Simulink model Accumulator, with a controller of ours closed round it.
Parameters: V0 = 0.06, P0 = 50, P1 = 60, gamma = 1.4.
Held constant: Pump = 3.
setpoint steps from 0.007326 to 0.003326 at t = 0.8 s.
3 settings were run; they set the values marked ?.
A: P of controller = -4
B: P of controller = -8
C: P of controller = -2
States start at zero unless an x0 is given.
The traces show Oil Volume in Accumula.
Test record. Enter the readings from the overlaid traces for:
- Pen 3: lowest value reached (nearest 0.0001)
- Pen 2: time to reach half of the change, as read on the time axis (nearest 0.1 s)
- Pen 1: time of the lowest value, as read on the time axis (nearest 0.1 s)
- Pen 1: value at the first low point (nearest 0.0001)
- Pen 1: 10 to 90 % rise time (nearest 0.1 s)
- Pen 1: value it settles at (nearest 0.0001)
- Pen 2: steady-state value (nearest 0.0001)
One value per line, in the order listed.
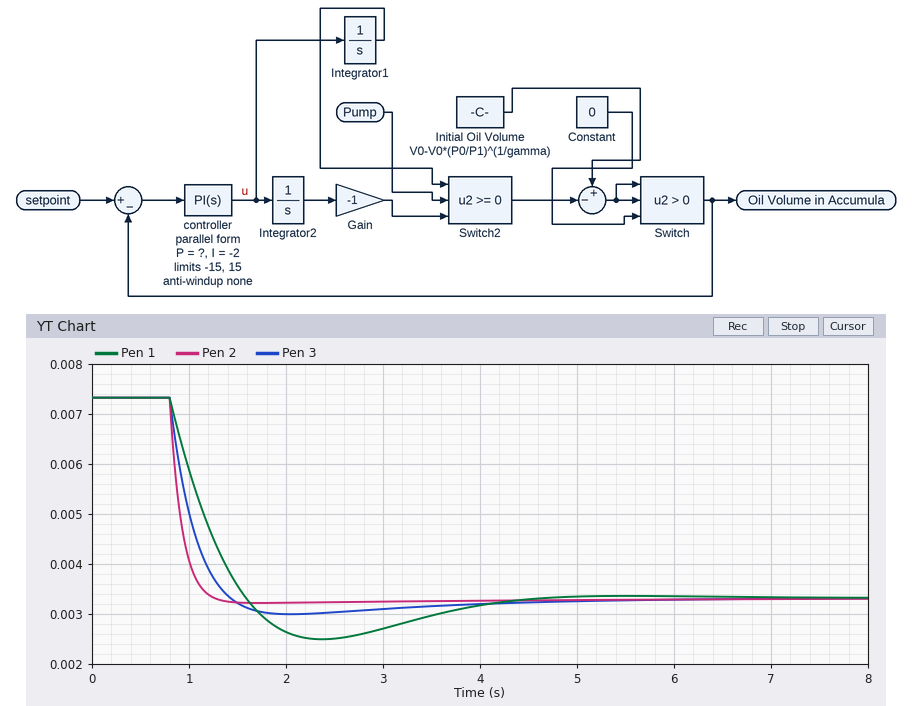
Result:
0.0030
0.9 s
2.4 s
0.0025
0.6 s
0.0033
0.0033
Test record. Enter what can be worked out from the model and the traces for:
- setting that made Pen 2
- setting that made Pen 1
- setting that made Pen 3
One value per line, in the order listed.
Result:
B
C
A
